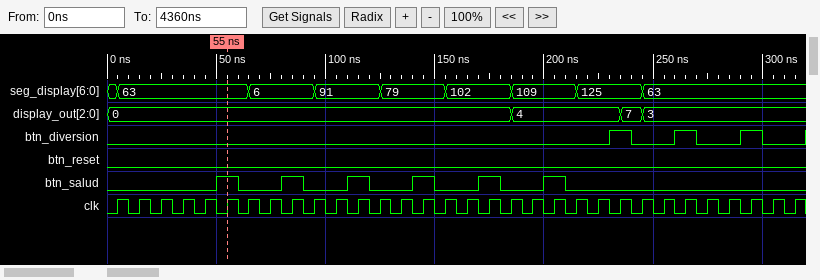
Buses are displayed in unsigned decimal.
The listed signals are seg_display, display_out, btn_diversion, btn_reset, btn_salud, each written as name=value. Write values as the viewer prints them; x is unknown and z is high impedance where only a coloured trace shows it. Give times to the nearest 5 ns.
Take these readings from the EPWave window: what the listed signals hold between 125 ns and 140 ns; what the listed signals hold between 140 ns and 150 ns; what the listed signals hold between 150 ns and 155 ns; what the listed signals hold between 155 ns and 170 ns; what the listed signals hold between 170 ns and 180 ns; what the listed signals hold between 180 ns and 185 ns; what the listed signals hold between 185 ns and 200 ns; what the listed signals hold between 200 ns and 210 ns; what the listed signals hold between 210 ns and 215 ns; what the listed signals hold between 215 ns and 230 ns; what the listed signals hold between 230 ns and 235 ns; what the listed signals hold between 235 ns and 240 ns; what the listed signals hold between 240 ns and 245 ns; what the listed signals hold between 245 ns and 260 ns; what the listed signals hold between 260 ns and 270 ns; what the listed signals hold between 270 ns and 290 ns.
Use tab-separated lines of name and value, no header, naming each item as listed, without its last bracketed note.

what the listed signals hold between 125 ns and 140 ns	seg_display=79, display_out=0, btn_diversion=0, btn_reset=0, btn_salud=0
what the listed signals hold between 140 ns and 150 ns	seg_display=79, display_out=0, btn_diversion=0, btn_reset=0, btn_salud=1
what the listed signals hold between 150 ns and 155 ns	seg_display=79, display_out=0, btn_diversion=0, btn_reset=0, btn_salud=0
what the listed signals hold between 155 ns and 170 ns	seg_display=102, display_out=0, btn_diversion=0, btn_reset=0, btn_salud=0
what the listed signals hold between 170 ns and 180 ns	seg_display=102, display_out=0, btn_diversion=0, btn_reset=0, btn_salud=1
what the listed signals hold between 180 ns and 185 ns	seg_display=102, display_out=0, btn_diversion=0, btn_reset=0, btn_salud=0
what the listed signals hold between 185 ns and 200 ns	seg_display=109, display_out=4, btn_diversion=0, btn_reset=0, btn_salud=0
what the listed signals hold between 200 ns and 210 ns	seg_display=109, display_out=4, btn_diversion=0, btn_reset=0, btn_salud=1
what the listed signals hold between 210 ns and 215 ns	seg_display=109, display_out=4, btn_diversion=0, btn_reset=0, btn_salud=0
what the listed signals hold between 215 ns and 230 ns	seg_display=125, display_out=4, btn_diversion=0, btn_reset=0, btn_salud=0
what the listed signals hold between 230 ns and 235 ns	seg_display=125, display_out=4, btn_diversion=1, btn_reset=0, btn_salud=0
what the listed signals hold between 235 ns and 240 ns	seg_display=125, display_out=7, btn_diversion=1, btn_reset=0, btn_salud=0
what the listed signals hold between 240 ns and 245 ns	seg_display=125, display_out=7, btn_diversion=0, btn_reset=0, btn_salud=0
what the listed signals hold between 245 ns and 260 ns	seg_display=63, display_out=3, btn_diversion=0, btn_reset=0, btn_salud=0
what the listed signals hold between 260 ns and 270 ns	seg_display=63, display_out=3, btn_diversion=1, btn_reset=0, btn_salud=0
what the listed signals hold between 270 ns and 290 ns	seg_display=63, display_out=3, btn_diversion=0, btn_reset=0, btn_salud=0
